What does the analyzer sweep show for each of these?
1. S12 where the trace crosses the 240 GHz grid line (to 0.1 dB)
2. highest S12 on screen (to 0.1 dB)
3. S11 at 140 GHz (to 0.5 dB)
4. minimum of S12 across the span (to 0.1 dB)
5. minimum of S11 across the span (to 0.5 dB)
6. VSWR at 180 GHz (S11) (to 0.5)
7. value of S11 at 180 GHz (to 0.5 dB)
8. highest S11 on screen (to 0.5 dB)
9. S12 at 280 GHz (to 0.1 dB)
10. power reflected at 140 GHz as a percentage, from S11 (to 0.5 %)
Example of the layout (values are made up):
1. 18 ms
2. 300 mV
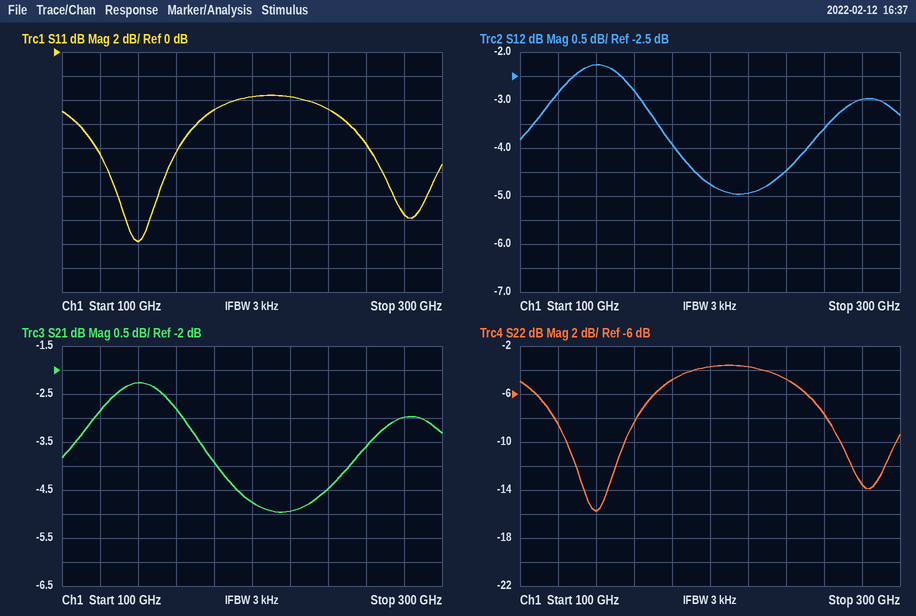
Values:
1. -4.5 dB
2. -2.3 dB
3. -16.0 dB
4. -5.0 dB
5. -16.0 dB
6. 3.5
7. -5.0 dB
8. -3.5 dB
9. -3.0 dB
10. 2.5 %
